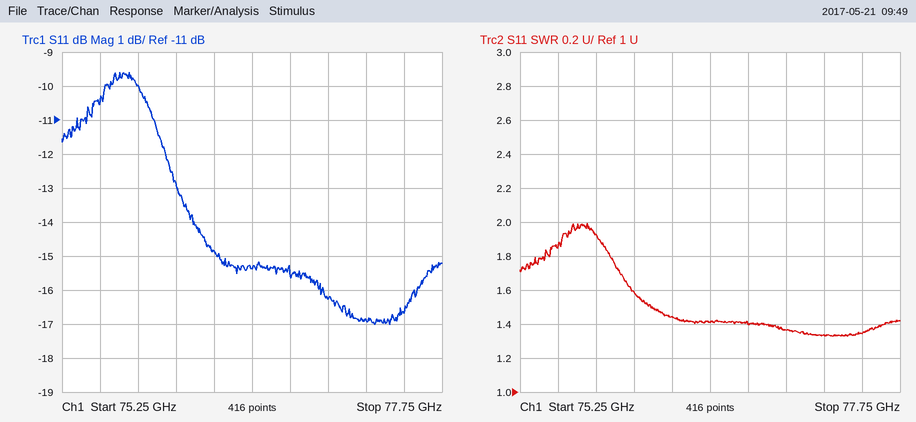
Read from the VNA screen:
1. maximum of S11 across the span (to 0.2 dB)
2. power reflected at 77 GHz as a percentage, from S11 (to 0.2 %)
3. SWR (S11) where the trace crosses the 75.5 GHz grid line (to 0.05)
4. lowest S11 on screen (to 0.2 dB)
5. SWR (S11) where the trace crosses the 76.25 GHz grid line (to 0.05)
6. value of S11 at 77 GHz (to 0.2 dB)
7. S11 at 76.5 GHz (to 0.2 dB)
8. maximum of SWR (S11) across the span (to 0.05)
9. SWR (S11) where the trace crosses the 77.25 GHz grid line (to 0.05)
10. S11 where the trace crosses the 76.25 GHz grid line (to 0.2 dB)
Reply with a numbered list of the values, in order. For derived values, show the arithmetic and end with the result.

1. -9.6 dB
2. 10^(-16.2/10) ≈ 2.4 %
3. 1.85
4. -17.0 dB
5. 1.45
6. -16.2 dB
7. -15.4 dB
8. 2.00
9. 1.35
10. -14.8 dB
